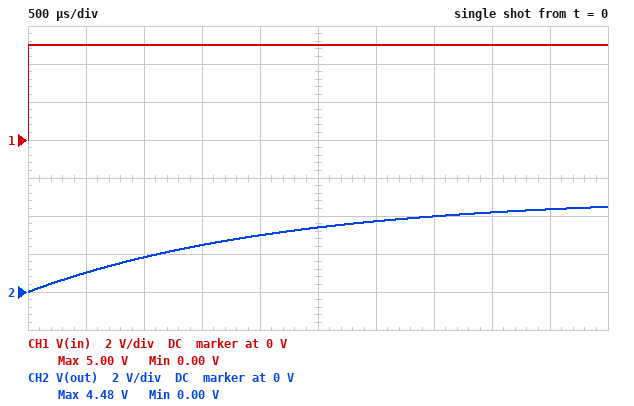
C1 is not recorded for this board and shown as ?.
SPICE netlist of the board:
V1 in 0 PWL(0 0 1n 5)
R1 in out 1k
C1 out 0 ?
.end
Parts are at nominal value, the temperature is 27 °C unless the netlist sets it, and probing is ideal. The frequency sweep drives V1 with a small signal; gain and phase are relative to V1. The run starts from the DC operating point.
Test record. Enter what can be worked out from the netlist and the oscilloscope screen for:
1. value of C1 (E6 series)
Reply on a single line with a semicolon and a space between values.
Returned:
2.2 µF
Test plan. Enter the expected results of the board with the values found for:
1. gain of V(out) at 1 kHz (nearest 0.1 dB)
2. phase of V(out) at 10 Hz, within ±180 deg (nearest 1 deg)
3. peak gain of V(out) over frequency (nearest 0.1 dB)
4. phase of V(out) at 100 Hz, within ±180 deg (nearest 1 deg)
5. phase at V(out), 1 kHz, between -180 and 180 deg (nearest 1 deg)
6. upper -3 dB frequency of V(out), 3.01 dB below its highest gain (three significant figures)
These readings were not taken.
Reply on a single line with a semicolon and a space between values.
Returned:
-22.8 dB; -8 deg; 0 dB; -54 deg; -86 deg; 72.3 Hz
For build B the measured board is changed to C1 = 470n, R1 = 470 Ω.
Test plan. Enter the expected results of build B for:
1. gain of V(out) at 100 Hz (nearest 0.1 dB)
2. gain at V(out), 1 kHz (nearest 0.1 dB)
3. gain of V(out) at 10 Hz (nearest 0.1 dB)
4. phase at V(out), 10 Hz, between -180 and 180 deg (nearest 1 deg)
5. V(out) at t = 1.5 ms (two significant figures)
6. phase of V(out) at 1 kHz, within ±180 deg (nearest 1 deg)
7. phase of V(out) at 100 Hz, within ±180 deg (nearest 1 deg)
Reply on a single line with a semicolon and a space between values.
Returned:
-0.1 dB; -4.7 dB; 0 dB; -1 deg; 5.0 V; -54 deg; -8 deg
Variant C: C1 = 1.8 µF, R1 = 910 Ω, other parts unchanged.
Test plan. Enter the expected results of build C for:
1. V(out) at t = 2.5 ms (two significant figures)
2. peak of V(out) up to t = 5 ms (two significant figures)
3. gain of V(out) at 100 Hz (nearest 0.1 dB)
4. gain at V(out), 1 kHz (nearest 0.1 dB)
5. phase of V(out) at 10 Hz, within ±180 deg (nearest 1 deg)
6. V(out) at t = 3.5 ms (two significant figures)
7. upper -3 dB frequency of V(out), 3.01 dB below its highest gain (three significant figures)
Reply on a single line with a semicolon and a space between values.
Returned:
3.9 V; 4.8 V; -3.1 dB; -20.3 dB; -6 deg; 4.4 V; 97.2 Hz
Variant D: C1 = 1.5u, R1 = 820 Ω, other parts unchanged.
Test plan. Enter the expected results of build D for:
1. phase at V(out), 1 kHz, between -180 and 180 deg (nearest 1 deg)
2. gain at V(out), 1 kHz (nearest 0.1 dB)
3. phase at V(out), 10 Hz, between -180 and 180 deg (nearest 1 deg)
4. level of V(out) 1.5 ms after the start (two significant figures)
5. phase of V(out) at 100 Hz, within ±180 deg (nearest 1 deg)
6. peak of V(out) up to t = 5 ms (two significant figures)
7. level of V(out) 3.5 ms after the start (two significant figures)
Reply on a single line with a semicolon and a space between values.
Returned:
-83 deg; -17.8 dB; -4 deg; 3.5 V; -38 deg; 4.9 V; 4.7 V
